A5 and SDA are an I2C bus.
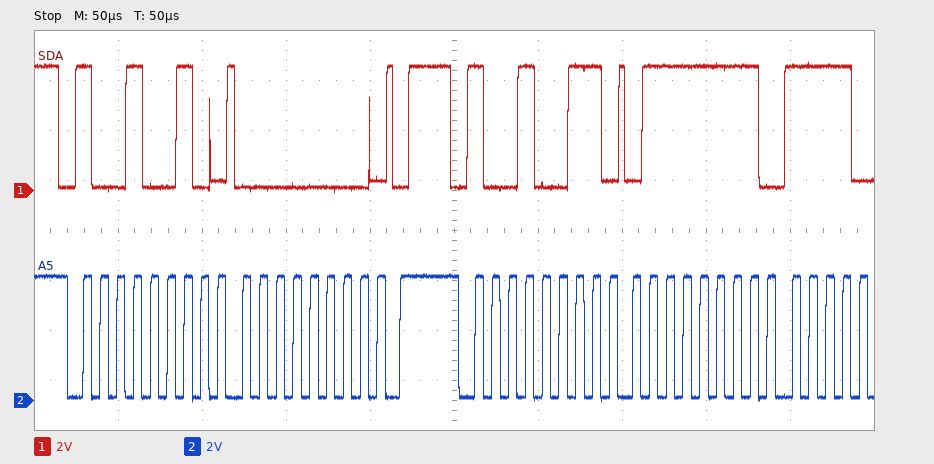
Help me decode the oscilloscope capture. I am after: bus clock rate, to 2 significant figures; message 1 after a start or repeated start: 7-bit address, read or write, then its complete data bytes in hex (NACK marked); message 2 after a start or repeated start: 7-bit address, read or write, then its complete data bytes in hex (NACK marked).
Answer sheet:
100 kHz
0x49 write: 00
0x49 read: 7F
